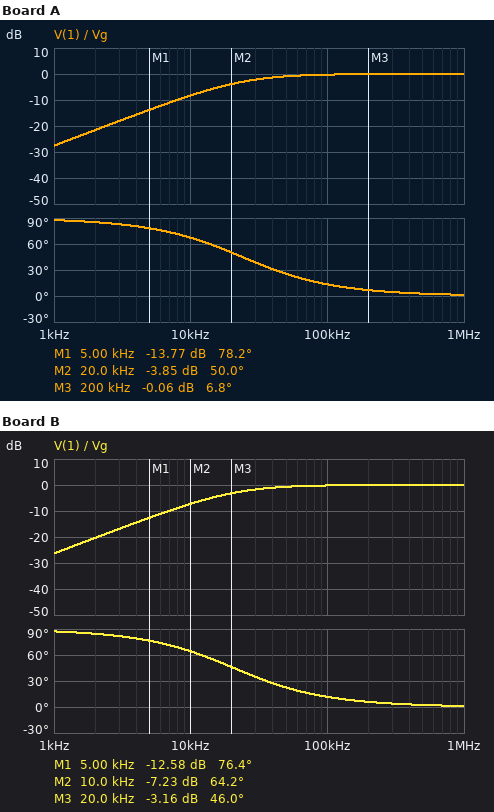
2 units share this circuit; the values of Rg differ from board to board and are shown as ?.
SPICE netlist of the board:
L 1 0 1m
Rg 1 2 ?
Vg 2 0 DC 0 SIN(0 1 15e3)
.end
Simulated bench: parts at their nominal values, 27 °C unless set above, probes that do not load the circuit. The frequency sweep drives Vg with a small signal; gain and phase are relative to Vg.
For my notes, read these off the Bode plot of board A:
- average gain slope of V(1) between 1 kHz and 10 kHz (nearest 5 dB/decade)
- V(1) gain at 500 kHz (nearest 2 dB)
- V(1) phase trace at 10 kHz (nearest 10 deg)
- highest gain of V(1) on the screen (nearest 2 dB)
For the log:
20 dB/decade
0 dB
70 deg
0 dB
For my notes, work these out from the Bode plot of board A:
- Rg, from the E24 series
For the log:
150 Ω
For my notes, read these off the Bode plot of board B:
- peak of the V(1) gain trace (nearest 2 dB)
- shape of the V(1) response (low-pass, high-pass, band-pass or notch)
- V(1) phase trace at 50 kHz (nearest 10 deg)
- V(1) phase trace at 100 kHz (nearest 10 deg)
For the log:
0 dB
high-pass
20 deg
10 deg
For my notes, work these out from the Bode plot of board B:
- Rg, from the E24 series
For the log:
130 Ω
